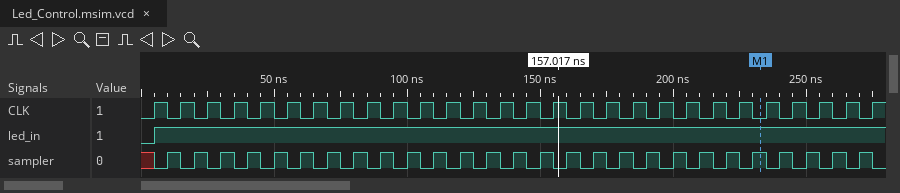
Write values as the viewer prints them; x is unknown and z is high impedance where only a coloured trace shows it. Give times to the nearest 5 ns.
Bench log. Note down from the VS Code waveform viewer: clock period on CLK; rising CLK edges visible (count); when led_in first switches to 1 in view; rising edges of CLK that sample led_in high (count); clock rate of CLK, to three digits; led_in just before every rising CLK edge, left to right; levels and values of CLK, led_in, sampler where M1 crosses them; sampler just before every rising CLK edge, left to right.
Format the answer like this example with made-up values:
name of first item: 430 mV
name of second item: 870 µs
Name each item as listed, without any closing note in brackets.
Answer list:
clock period on CLK: 10 ns
rising CLK edges visible: 28
when led_in first switches to 1 in view: 5 ns
rising edges of CLK that sample led_in high: 27
clock rate of CLK, to three digits: 100 MHz
led_in just before every rising CLK edge, left to right: 0 1 1 1 1 1 1 1 1 1 1 1 1 1 1 1 1 1 1 1 1 1 1 1 1 1 1 1
levels and values of CLK, led_in, sampler where M1 crosses them: CLK=0, led_in=1, sampler=1
sampler just before every rising CLK edge, left to right: x 1 1 1 1 1 1 1 1 1 1 1 1 1 1 1 1 1 1 1 1 1 1 1 1 1 1 1
